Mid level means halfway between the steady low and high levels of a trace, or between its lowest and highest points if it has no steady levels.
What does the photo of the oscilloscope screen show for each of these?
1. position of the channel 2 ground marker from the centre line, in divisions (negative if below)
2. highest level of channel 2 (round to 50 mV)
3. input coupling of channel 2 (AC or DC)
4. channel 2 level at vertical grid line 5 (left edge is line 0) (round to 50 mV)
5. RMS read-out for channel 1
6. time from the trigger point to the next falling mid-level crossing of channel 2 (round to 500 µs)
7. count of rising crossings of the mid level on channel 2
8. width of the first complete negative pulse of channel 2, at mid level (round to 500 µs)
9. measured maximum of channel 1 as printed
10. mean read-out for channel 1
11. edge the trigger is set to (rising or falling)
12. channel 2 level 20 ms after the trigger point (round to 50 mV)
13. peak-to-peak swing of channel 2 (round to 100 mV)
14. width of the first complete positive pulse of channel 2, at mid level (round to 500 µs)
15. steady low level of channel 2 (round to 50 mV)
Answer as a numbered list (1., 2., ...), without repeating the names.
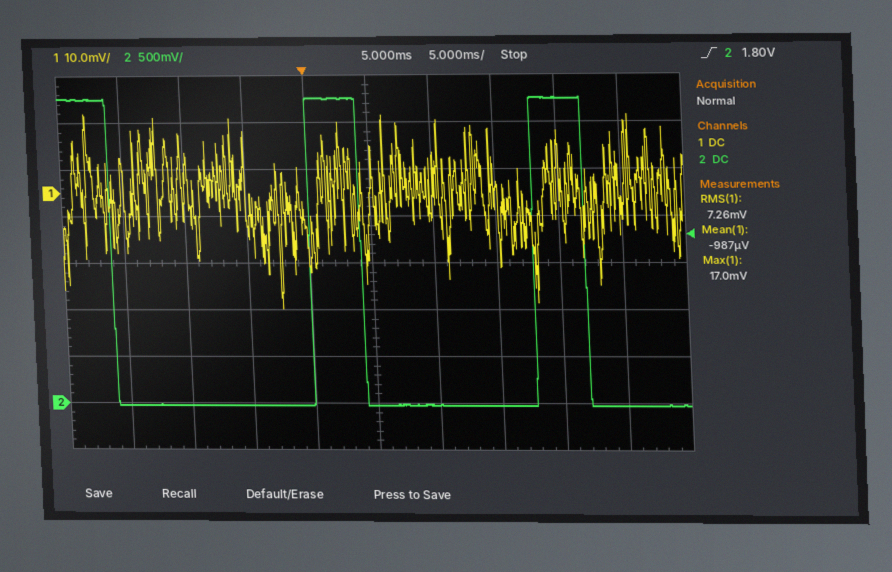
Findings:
1. -3.0 div
2. 3.25 V
3. DC
4. 0 mV
5. 7.26 mV
6. 4.0 ms
7. 2
8. 16.0 ms
9. 17.0 mV
10. -987 µV
11. rising
12. 3.25 V
13. 3.30 V
14. 4.0 ms
15. 0 mV
